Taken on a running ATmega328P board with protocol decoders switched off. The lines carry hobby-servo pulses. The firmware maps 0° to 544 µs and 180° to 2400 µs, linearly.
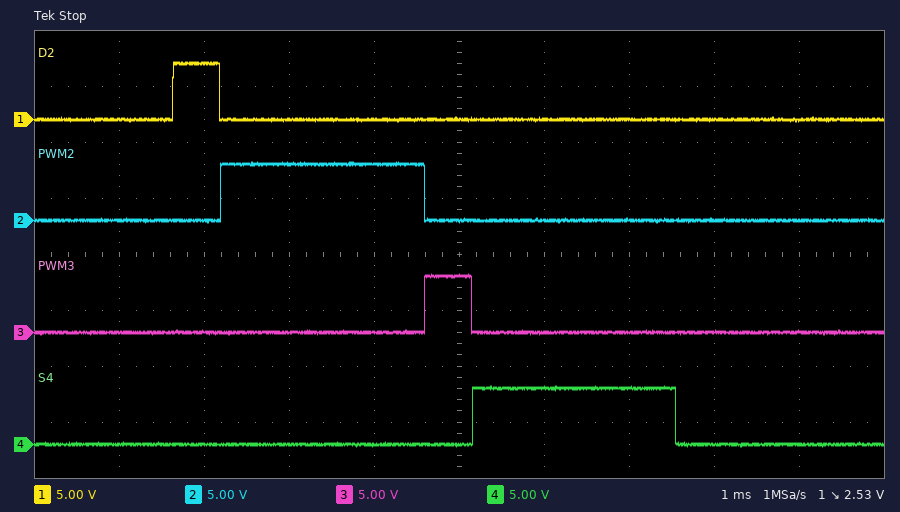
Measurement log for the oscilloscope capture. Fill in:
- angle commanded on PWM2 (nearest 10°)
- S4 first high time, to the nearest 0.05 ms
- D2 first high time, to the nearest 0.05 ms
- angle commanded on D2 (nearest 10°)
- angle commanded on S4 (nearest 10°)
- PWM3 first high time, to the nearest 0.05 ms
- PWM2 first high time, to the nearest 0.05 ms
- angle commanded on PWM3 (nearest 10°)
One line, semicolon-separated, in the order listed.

180°; 2.40 ms; 0.55 ms; 0°; 180°; 0.55 ms; 2.40 ms; 0°
